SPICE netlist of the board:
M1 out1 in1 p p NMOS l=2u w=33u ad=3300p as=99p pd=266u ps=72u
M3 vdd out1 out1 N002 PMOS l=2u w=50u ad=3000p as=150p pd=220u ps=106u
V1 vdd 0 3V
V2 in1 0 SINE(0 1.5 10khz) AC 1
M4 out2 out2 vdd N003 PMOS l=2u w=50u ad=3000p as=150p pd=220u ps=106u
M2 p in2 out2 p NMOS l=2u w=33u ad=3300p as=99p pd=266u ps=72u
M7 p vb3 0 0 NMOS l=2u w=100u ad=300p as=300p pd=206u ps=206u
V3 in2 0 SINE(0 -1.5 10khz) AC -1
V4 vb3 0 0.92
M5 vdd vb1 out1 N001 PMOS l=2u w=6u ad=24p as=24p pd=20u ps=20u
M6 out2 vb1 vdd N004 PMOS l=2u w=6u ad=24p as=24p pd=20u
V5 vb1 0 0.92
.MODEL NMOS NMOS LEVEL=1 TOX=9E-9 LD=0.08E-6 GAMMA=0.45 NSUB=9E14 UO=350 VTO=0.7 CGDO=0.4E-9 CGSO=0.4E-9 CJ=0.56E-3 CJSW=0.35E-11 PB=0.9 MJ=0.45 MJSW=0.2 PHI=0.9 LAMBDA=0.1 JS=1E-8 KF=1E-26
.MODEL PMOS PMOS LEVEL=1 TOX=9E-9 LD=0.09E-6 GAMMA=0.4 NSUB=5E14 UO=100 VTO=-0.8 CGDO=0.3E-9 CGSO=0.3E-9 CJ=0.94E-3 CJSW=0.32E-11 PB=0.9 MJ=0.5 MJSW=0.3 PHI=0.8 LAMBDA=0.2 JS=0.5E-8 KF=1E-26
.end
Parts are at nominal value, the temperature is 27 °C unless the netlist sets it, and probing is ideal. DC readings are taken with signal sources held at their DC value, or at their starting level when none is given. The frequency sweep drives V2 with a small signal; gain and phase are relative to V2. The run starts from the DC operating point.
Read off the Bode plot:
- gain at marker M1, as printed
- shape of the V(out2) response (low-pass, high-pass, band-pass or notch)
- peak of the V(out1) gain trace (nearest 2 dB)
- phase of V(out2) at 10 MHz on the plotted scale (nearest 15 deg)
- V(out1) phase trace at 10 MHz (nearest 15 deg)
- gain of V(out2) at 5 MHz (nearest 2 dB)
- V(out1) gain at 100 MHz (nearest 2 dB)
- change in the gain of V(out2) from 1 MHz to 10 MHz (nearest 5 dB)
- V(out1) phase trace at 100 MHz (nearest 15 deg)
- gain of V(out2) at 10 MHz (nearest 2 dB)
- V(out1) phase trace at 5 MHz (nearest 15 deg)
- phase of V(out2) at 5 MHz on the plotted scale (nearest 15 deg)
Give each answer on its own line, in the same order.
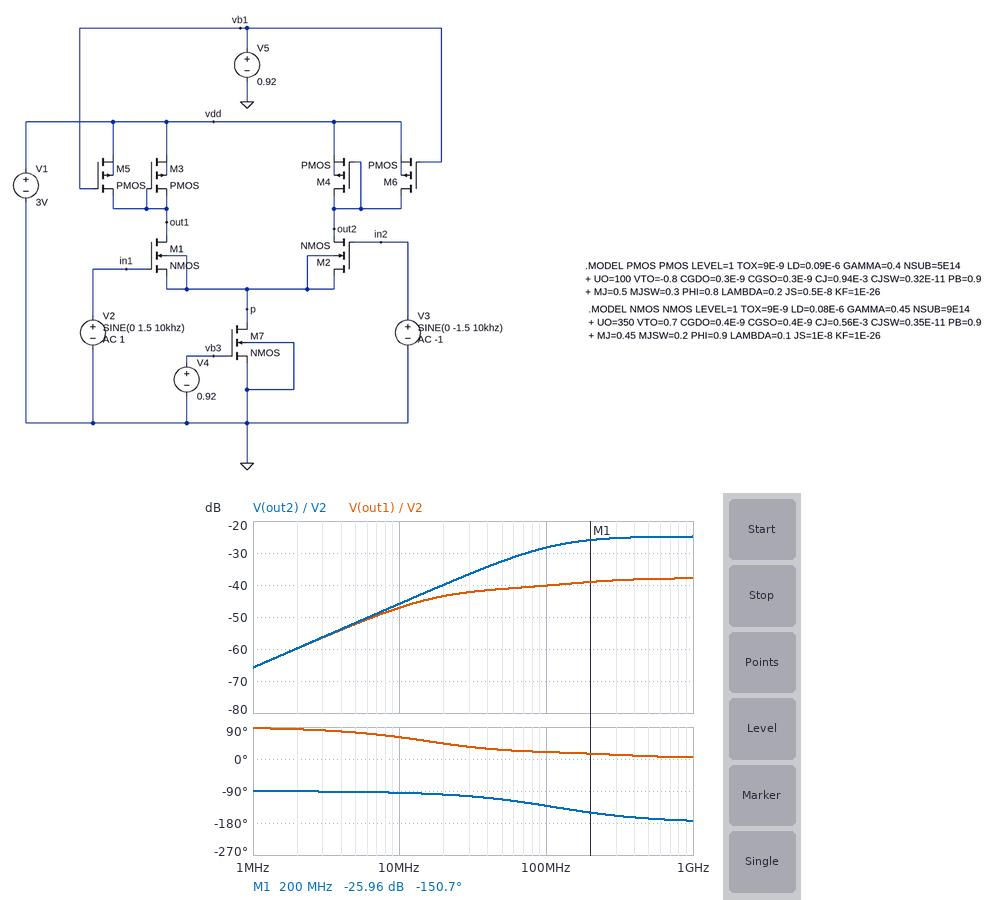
-25.96 dB
high-pass
-38 dB
-90 deg
60 deg
-52 dB
-40 dB
20 dB
15 deg
-46 dB
75 deg
-90 deg
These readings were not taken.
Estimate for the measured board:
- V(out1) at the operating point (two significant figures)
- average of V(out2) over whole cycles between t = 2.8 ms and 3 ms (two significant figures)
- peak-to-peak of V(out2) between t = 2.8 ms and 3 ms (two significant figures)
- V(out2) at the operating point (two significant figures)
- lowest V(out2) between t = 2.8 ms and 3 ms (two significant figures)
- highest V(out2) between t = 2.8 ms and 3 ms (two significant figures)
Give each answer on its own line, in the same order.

3.0 V
2.7 V
980 mV
3.0 V
2.0 V
3.0 V
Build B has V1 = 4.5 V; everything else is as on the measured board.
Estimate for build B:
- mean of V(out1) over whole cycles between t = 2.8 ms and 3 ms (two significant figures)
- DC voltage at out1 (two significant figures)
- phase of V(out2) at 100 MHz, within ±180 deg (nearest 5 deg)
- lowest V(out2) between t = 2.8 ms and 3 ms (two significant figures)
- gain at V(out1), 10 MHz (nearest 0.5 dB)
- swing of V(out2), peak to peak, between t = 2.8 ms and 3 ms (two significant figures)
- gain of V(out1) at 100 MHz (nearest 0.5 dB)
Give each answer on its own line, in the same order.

4.4 V
4.5 V
-110 deg
4.0 V
-53.0 dB
510 mV
-40.5 dB
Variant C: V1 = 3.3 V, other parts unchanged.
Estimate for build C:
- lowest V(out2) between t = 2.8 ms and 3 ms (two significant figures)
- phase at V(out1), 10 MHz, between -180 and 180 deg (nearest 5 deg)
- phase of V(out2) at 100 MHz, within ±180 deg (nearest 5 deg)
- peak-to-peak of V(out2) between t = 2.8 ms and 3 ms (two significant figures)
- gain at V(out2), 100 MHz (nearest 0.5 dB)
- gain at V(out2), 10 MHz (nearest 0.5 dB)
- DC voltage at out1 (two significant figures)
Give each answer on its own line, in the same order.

2.4 V
65 deg
-125 deg
880 mV
-29.5 dB
-47.5 dB
3.3 V
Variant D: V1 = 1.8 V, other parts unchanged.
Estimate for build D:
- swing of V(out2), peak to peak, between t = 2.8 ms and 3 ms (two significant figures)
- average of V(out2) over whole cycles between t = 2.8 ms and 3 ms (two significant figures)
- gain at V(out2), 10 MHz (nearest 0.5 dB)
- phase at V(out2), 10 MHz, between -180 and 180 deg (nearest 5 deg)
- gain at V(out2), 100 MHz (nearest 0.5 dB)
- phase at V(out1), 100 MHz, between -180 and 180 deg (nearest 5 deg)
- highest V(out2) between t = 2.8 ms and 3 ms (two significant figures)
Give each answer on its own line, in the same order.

1.2 V
1.4 V
-26.5 dB
-145 deg
-25.0 dB
10 deg
1.8 V
